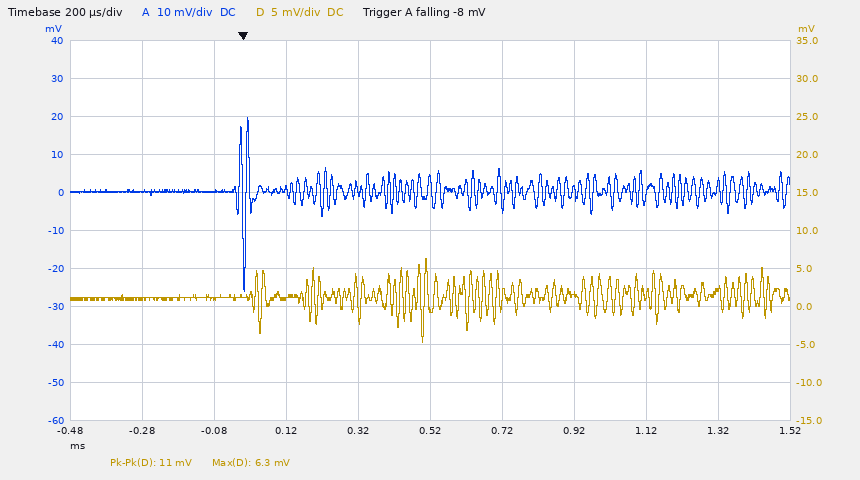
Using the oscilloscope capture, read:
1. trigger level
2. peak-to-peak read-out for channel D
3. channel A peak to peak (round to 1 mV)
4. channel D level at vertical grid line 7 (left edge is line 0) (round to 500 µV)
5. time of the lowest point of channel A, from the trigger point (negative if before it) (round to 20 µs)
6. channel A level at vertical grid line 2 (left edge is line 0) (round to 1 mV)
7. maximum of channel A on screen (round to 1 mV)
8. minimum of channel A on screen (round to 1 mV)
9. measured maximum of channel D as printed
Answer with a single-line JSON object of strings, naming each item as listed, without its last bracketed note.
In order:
{"trigger level": "-8 mV", "peak-to-peak read-out for channel D": "11 mV", "channel A peak to peak": "46 mV", "channel D level at vertical grid line 7 (left edge is line 0)": "1.5 mV", "time of the lowest point of channel A, from the trigger point (negative if before it)": "0 µs", "channel A level at vertical grid line 2 (left edge is line 0)": "0 mV", "maximum of channel A on screen": "20 mV", "minimum of channel A on screen": "-26 mV", "measured maximum of channel D as printed": "6.3 mV"}
